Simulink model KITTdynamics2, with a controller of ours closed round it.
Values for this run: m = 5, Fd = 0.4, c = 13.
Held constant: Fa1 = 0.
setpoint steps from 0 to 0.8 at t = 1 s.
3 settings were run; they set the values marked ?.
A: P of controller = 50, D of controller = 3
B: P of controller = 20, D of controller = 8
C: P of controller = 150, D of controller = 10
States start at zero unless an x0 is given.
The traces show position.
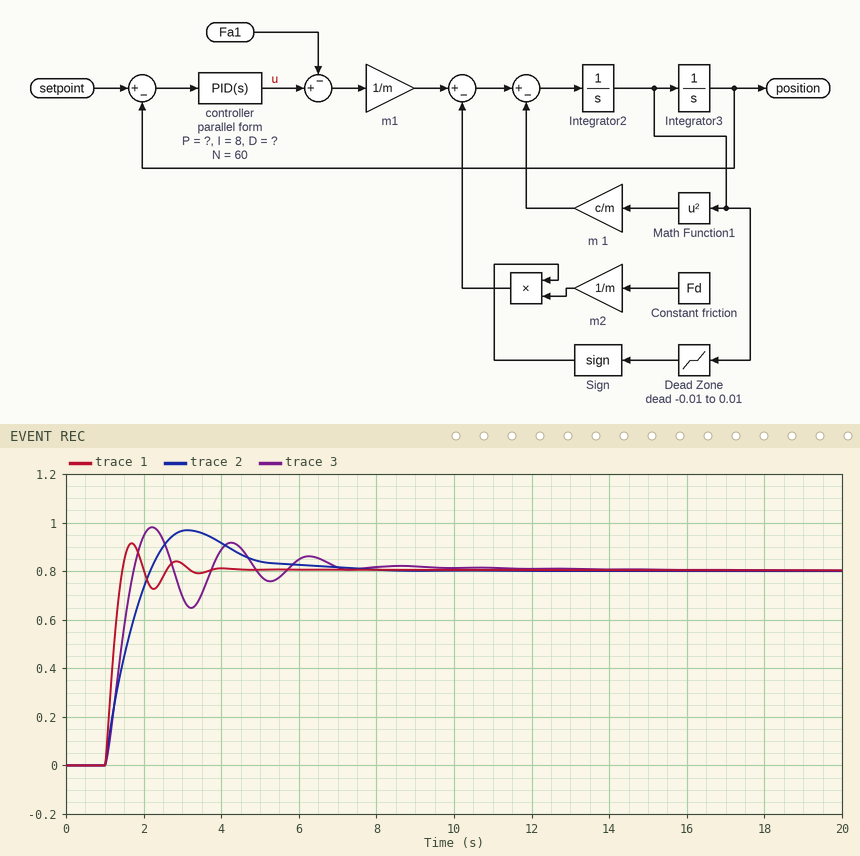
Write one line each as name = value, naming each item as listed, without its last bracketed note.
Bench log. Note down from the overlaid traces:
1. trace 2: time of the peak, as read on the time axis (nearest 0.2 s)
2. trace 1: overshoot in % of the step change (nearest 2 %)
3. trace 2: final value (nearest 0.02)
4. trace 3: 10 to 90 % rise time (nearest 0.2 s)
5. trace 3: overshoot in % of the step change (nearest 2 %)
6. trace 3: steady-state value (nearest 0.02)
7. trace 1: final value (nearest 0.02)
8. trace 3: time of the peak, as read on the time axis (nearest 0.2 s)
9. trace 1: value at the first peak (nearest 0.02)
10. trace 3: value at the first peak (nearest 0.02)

trace 2: time of the peak, as read on the time axis = 3.2 s
trace 1: overshoot in % of the step change = 14 %
trace 2: final value = 0.80
trace 3: 10 to 90 % rise time = 0.6 s
trace 3: overshoot in % of the step change = 22 %
trace 3: steady-state value = 0.80
trace 1: final value = 0.80
trace 3: time of the peak, as read on the time axis = 2.2 s
trace 1: value at the first peak = 0.92
trace 3: value at the first peak = 0.98
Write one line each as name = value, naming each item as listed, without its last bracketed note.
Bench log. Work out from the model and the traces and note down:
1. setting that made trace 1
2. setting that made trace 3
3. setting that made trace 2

setting that made trace 1 = C
setting that made trace 3 = A
setting that made trace 2 = B
